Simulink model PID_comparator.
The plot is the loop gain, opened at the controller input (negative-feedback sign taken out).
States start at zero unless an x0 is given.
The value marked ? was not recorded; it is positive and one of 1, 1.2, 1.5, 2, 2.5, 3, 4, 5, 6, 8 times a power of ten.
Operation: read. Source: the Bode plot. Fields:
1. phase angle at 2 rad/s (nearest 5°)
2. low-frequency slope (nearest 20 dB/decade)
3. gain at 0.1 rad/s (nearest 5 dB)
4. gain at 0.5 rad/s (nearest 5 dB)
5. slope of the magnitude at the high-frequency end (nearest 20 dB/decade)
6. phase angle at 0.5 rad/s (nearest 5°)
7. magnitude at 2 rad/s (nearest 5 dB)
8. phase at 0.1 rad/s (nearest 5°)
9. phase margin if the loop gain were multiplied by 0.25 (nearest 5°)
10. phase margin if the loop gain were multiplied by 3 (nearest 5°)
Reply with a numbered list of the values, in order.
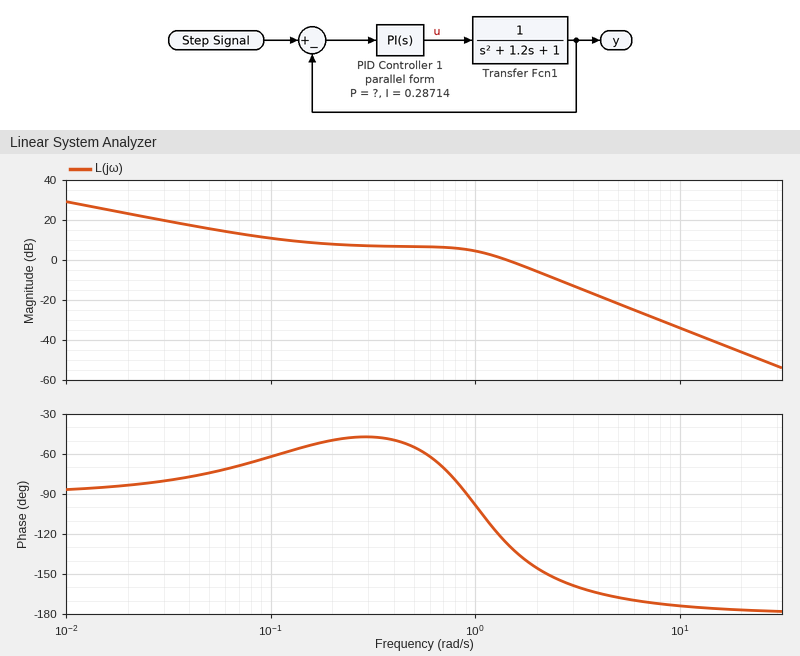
1. -145°
2. -20 dB/decade
3. 10 dB
4. 5 dB
5. -40 dB/decade
6. -55°
7. -5 dB
8. -60°
9. 115°
10. 25°
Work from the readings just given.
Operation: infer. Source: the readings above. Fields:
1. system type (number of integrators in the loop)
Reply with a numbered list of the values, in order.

1. 1
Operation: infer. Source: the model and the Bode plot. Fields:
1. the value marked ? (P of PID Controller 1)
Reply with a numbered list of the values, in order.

1. 2
